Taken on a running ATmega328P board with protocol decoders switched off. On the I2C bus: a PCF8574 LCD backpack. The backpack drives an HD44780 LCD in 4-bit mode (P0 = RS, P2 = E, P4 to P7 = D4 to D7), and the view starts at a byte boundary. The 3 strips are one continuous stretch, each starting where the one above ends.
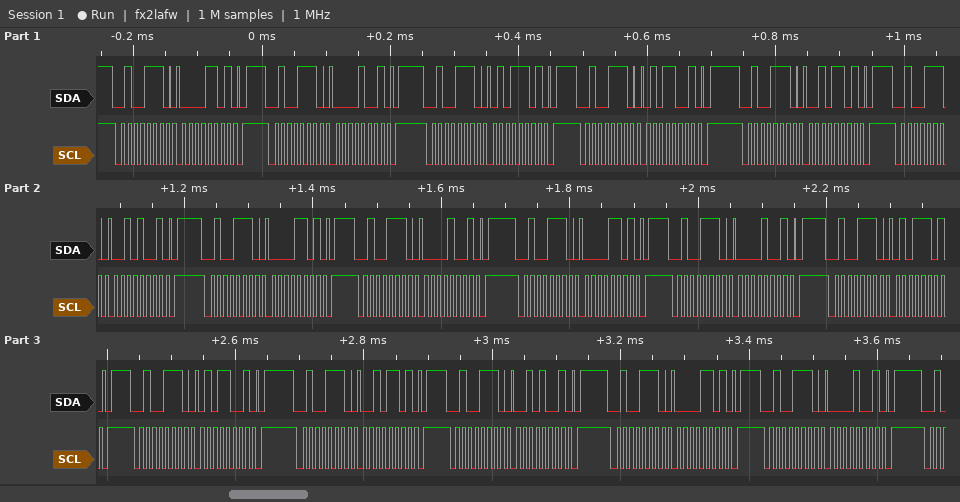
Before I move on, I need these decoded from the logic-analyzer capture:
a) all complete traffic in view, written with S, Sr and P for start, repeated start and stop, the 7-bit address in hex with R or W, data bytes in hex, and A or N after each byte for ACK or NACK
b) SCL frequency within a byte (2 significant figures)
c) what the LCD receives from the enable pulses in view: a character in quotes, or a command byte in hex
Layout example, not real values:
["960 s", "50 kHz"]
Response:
["S 27W A 0D A P S 27W A 09 A P S 27W A 5D A P S 27W A 59 A P S 27W A 2D A P S 27W A 29 A P S 27W A 0D A P S 27W A 09 A P S 27W A 0D A P S 27W A 09 A P S 27W A 5D A P S 27W A 59 A P S 27W A 2D A P S 27W A 29 A P S 27W A 0D A P S 27W A 09 A P", "100 kHz", "data 0x05 ' ' data 0x05 ' '"]
